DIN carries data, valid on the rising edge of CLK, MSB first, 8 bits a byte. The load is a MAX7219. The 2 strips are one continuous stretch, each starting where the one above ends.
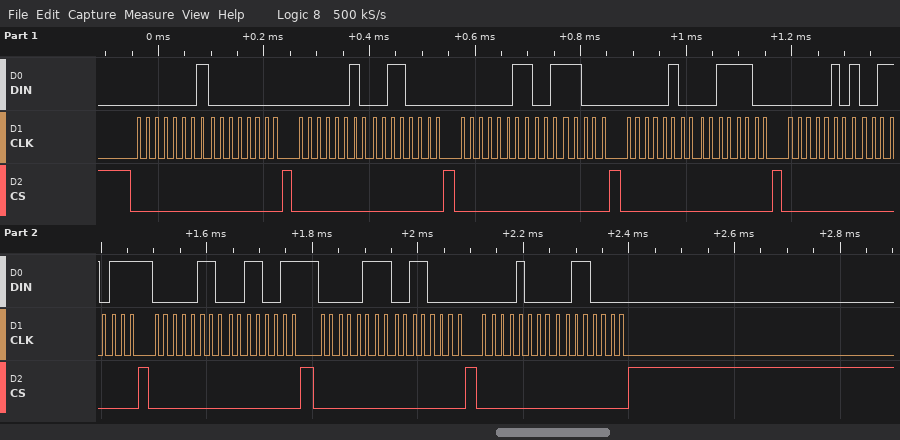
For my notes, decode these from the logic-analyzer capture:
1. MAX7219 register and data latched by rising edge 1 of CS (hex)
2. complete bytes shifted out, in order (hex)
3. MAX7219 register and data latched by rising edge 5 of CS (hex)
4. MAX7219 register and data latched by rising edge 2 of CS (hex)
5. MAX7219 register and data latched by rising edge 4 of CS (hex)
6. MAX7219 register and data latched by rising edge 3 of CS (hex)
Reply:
register 0x1, data 0x00
0x01 0x00 0x02 0x30 0x03 0x38 0x04 0x3C 0x05 0x37 0x06 0x33 0x07 0x30 0x08 0x30
register 0x5, data 0x37
register 0x2, data 0x30
register 0x4, data 0x3C
register 0x3, data 0x38
